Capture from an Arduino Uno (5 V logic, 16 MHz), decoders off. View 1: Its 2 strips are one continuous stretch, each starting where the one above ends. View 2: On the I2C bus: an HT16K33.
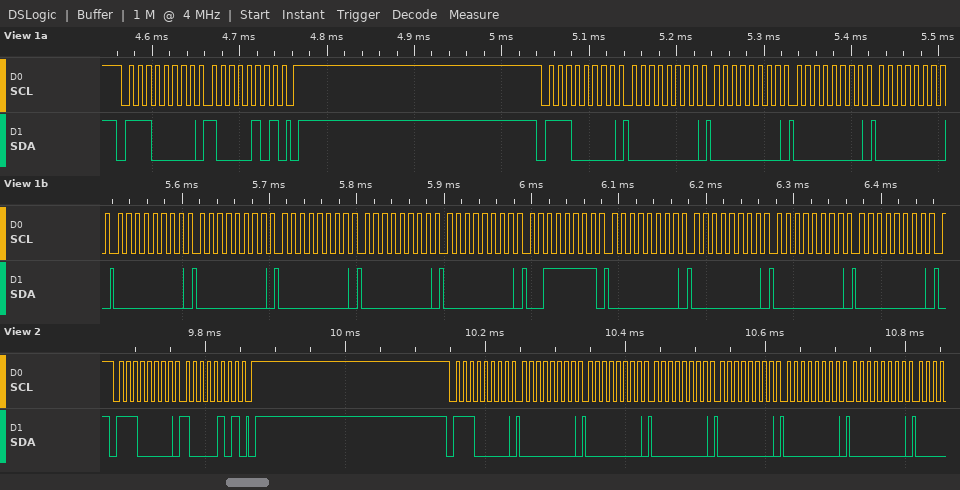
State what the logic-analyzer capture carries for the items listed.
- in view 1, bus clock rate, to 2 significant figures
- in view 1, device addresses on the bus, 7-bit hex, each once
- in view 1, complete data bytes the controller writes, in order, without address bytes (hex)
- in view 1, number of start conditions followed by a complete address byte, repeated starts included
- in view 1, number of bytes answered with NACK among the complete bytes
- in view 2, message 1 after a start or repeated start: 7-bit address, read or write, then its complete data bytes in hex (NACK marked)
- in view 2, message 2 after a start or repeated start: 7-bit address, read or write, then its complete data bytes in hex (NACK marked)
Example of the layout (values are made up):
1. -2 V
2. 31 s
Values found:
1. 100 kHz
2. 0x70
3. 85 00 00 00 00 00 00 00 00 00 3F 00 00 00 00
4. 2
5. 0
6. 0x70 write: 85
7. 0x70 write: 00 00 00 00 00 00
